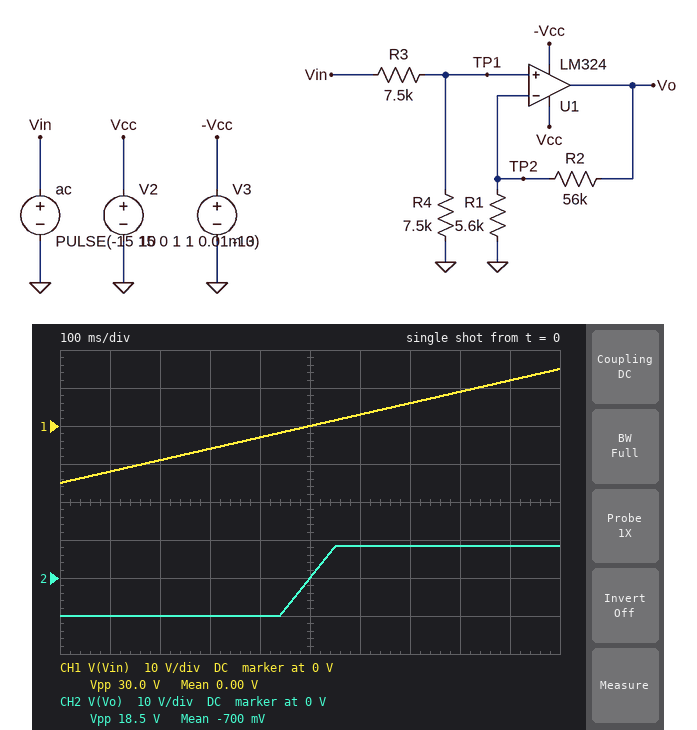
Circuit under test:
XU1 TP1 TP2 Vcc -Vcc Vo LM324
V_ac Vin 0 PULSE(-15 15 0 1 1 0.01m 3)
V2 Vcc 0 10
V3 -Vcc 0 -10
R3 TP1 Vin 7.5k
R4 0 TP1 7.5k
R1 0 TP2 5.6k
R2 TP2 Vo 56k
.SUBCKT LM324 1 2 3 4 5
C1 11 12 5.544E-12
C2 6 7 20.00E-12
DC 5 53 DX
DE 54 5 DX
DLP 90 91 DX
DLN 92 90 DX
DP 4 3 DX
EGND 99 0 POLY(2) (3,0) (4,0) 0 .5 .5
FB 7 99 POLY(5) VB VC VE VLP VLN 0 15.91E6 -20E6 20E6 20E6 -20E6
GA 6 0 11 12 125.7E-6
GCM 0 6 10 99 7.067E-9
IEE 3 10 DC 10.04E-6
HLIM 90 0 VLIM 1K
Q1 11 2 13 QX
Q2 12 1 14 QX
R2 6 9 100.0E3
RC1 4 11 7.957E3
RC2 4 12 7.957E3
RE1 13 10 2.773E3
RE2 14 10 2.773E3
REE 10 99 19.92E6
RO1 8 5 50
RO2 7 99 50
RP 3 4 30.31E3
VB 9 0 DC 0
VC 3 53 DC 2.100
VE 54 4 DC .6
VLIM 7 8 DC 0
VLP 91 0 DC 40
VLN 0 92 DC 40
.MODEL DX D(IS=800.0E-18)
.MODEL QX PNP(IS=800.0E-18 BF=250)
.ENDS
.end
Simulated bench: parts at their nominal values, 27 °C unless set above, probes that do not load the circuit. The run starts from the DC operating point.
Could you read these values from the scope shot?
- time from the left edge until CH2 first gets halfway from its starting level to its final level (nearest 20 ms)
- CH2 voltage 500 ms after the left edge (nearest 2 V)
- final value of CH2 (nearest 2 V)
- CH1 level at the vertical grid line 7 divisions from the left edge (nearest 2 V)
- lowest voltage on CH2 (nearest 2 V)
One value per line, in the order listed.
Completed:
500 ms
0 V
8 V
6 V
-10 V
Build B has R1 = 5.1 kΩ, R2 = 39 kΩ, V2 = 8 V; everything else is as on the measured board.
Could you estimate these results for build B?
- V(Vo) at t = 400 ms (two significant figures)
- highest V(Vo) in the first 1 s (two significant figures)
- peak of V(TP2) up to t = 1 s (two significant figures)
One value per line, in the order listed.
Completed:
-10 V
6.5 V
750 mV
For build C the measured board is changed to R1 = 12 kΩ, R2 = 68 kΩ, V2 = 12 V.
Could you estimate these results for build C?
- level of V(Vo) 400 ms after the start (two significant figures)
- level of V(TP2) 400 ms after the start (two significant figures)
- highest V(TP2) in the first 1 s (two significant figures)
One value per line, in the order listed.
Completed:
-9.9 V
-1.5 V
1.6 V
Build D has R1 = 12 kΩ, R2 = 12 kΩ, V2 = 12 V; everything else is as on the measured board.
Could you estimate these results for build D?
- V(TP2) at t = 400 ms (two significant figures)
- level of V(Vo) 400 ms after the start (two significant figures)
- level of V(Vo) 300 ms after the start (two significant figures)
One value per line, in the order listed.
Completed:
-1.5 V
-3.0 V
-6.0 V
